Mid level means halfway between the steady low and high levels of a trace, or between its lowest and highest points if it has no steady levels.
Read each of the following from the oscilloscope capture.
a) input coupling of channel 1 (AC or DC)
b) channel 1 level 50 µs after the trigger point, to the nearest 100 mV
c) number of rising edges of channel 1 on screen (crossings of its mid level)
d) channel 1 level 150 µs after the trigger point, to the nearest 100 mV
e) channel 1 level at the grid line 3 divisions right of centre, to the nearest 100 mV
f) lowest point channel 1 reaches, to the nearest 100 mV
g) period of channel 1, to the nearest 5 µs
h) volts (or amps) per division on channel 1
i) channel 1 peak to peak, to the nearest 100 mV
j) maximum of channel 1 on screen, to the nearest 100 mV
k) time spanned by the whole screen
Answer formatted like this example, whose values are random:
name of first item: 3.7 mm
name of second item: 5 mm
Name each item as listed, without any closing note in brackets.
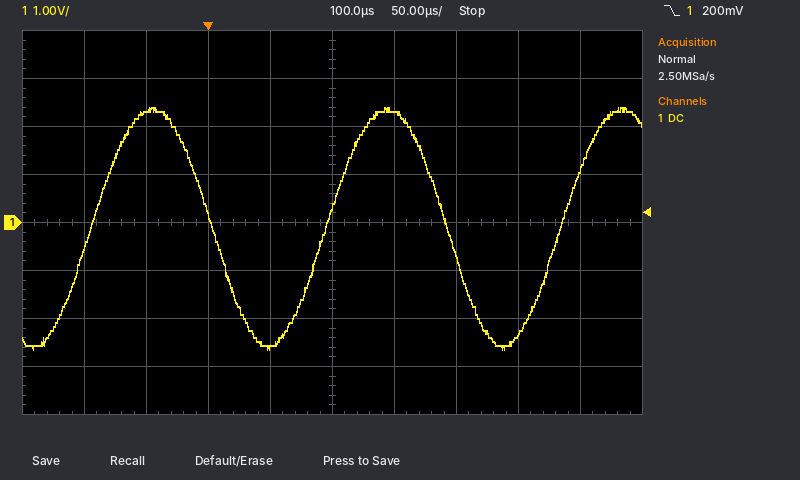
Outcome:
input coupling of channel 1: DC
channel 1 level 50 µs after the trigger point, to the nearest 100 mV: -2.6 V
number of rising edges of channel 1 on screen: 3
channel 1 level 150 µs after the trigger point, to the nearest 100 mV: 2.3 V
channel 1 level at the grid line 3 divisions right of centre, to the nearest 100 mV: -2.3 V
lowest point channel 1 reaches, to the nearest 100 mV: -2.6 V
period of channel 1, to the nearest 5 µs: 190 µs
volts (or amps) per division on channel 1: 1 V
channel 1 peak to peak, to the nearest 100 mV: 5.0 V
maximum of channel 1 on screen, to the nearest 100 mV: 2.4 V
time spanned by the whole screen: 500 µs
